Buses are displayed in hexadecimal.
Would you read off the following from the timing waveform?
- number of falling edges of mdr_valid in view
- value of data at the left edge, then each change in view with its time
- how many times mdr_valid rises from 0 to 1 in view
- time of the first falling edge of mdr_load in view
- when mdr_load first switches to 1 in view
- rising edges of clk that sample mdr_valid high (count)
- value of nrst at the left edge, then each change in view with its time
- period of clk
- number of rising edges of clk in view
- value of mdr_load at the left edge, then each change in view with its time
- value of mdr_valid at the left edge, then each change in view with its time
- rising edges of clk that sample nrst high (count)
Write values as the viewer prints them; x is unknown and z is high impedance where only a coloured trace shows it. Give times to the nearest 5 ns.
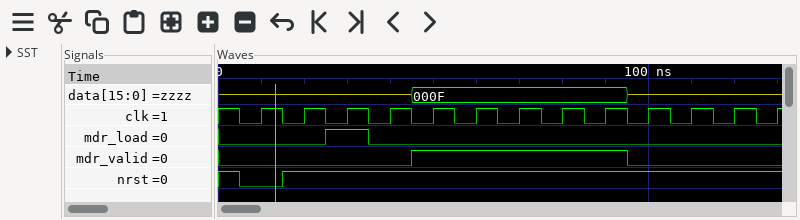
1
z, 000F at 45 ns, z at 95 ns
1
35 ns
25 ns
5
1, 0 at 5 ns, 1 at 15 ns
10 ns
13
0, 1 at 25 ns, 0 at 35 ns
0, 1 at 45 ns, 0 at 95 ns
12
